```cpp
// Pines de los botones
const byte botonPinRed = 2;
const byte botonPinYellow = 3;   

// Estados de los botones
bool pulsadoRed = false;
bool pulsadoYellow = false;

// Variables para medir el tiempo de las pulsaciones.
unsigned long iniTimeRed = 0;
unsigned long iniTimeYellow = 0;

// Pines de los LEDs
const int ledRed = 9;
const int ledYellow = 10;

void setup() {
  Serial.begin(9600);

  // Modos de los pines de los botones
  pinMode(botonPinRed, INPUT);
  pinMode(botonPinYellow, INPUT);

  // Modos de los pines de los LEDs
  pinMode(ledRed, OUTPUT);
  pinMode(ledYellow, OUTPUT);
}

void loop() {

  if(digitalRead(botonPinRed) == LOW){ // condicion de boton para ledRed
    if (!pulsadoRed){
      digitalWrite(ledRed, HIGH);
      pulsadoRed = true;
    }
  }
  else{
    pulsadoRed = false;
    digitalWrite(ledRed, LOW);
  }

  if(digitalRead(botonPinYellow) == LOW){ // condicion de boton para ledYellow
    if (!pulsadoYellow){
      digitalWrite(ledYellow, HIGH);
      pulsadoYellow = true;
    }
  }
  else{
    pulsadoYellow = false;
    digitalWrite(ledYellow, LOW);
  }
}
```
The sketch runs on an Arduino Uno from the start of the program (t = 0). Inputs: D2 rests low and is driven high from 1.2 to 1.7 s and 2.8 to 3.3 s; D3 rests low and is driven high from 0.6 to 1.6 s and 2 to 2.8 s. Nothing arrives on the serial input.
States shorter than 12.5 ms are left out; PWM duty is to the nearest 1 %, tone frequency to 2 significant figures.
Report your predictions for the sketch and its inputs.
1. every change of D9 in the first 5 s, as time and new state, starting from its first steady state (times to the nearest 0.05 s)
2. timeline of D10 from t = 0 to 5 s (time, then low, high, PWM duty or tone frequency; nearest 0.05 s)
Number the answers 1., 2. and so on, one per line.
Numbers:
1. 0 s high; 1.2 s low; 1.7 s high; 2.8 s low; 3.3 s high
2. 0 s high; 0.6 s low; 1.6 s high; 2 s low; 2.8 s high
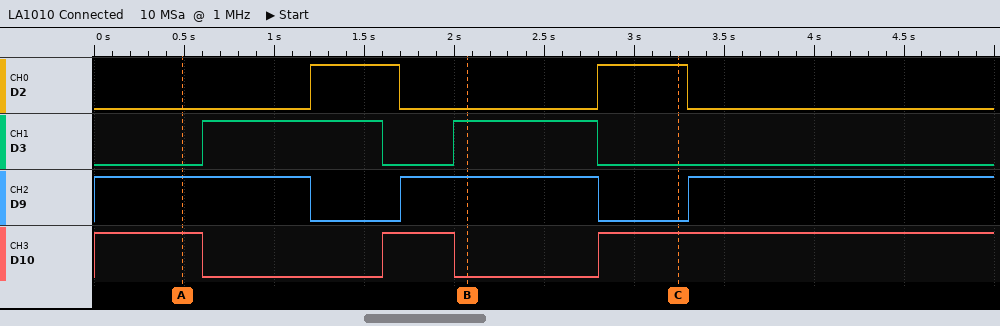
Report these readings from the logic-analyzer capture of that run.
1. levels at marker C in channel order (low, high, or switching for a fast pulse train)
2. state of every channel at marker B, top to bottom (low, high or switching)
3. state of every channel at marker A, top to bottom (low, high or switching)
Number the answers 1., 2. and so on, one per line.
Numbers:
1. D2 high, D3 low, D9 low, D10 high
2. D2 low, D3 high, D9 high, D10 low
3. D2 low, D3 low, D9 high, D10 high
